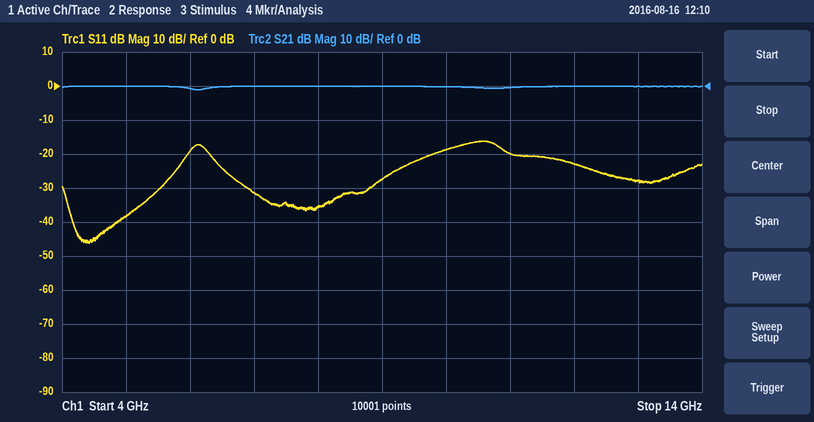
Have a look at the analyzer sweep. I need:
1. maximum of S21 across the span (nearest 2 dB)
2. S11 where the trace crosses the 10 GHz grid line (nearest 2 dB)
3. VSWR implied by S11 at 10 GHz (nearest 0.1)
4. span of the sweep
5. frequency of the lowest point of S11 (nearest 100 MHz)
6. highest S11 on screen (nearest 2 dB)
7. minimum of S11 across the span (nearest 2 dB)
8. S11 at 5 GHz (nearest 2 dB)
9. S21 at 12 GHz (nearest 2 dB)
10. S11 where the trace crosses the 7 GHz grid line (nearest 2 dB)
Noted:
0 dB
-18 dB
1.3
10 GHz
4.4 GHz
-16 dB
-46 dB
-38 dB
0 dB
-32 dB
